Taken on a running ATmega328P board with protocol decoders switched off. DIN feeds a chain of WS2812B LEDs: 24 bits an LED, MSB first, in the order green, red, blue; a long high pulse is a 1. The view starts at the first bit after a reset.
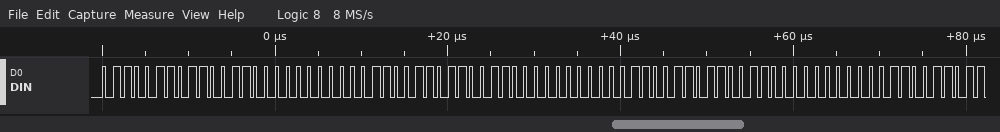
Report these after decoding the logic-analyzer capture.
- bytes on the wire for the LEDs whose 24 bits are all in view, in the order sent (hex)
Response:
66 CC 00 66 CC 00 66 CC 00
